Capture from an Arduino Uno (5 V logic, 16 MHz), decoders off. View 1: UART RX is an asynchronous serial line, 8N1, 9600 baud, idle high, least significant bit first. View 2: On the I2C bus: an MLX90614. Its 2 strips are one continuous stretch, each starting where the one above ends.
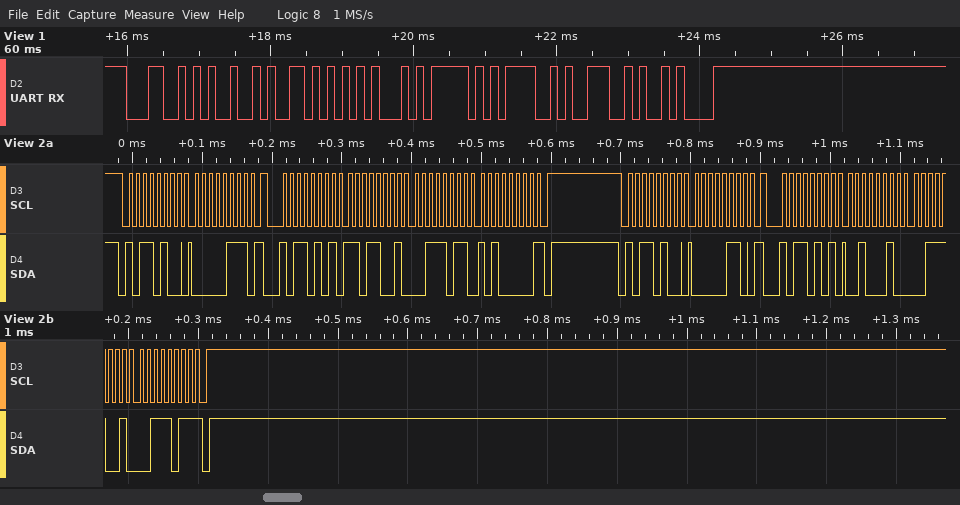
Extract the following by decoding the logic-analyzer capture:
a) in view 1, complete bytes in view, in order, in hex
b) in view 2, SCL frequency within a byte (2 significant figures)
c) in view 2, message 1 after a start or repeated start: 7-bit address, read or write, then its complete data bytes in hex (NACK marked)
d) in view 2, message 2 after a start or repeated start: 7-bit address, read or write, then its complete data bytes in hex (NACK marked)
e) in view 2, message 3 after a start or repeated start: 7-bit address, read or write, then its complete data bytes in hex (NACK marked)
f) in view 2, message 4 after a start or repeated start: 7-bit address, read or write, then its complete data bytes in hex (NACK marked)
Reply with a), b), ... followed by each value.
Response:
a) 4C 49 56 45 5F 4F 4E 0A
b) 100 kHz
c) 0x5A write: 07
d) 0x5A read: D9 3B A0 NACK
e) 0x5A write: 06
f) 0x5A read: 22 39 3B NACK
